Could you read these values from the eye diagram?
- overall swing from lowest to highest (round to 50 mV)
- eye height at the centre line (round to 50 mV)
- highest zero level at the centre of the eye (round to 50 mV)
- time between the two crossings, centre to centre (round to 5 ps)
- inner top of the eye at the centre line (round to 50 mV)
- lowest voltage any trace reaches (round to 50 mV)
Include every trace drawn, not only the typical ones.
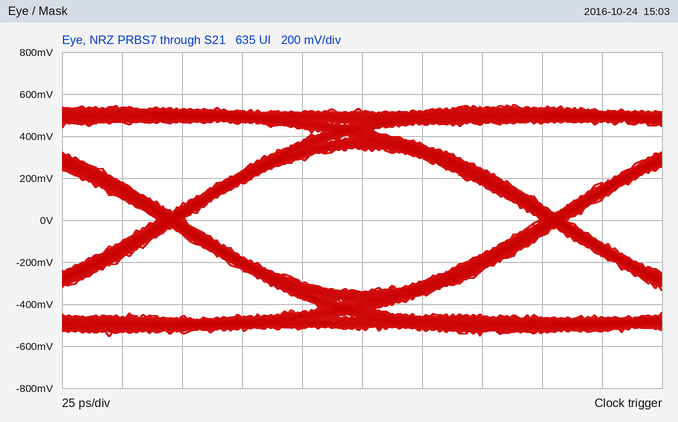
1.10 V
700 mV
-350 mV
160 ps
350 mV
-550 mV
